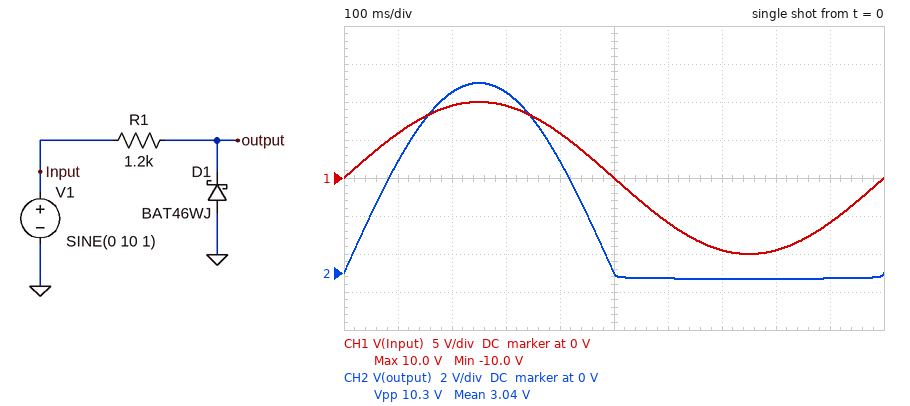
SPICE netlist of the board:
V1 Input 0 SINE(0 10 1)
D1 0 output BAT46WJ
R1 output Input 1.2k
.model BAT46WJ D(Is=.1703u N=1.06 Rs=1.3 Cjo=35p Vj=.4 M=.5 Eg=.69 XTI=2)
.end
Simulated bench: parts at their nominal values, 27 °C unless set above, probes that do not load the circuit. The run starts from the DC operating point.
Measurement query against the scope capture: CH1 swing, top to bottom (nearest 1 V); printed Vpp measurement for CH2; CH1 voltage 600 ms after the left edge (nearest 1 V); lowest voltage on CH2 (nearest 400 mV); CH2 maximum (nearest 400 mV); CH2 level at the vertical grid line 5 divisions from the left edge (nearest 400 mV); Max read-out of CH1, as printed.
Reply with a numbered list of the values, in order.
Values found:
1. 20 V
2. 10.3 V
3. -6 V
4. -400 mV
5. 10.0 V
6. 0 V
7. 10.0 V
